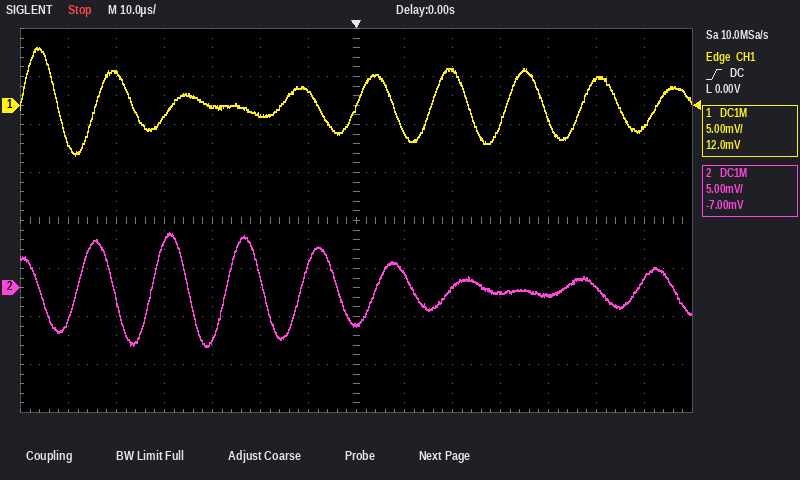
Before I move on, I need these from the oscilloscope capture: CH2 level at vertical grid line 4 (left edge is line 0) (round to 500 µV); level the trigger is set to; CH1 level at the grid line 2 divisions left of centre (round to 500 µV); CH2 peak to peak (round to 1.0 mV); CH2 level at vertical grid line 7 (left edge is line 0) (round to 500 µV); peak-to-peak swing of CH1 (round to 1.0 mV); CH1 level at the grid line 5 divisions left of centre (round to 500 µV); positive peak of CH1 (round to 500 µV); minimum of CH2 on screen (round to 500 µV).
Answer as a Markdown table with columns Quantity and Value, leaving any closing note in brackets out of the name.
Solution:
| Quantity | Value |
|---|---|
| CH2 level at vertical grid line 4 (left edge is line 0) | -5.5 mV |
| level the trigger is set to | 0.00 V |
| CH1 level at the grid line 2 divisions left of centre | -1.0 mV |
| CH2 peak to peak | 12.0 mV |
| CH2 level at vertical grid line 7 (left edge is line 0) | -4.0 mV |
| peak-to-peak swing of CH1 | 11.0 mV |
| CH1 level at the grid line 5 divisions left of centre | 3.5 mV |
| positive peak of CH1 | 6.0 mV |
| minimum of CH2 on screen | -6.0 mV |
